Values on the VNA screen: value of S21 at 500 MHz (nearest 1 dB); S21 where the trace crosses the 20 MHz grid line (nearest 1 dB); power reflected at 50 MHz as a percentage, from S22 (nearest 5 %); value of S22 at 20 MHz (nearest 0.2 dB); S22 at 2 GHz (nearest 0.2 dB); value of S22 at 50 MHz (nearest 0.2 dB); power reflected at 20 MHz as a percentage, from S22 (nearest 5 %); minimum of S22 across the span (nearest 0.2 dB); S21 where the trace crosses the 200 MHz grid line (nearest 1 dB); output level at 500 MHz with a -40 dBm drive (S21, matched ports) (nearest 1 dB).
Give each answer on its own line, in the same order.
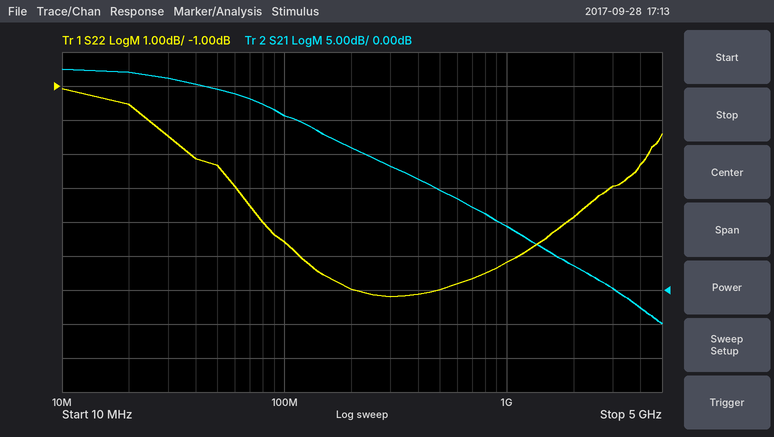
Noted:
15 dB
32 dB
45 %
-1.6 dB
-4.8 dB
-3.4 dB
70 %
-7.2 dB
21 dB
-25 dBm
